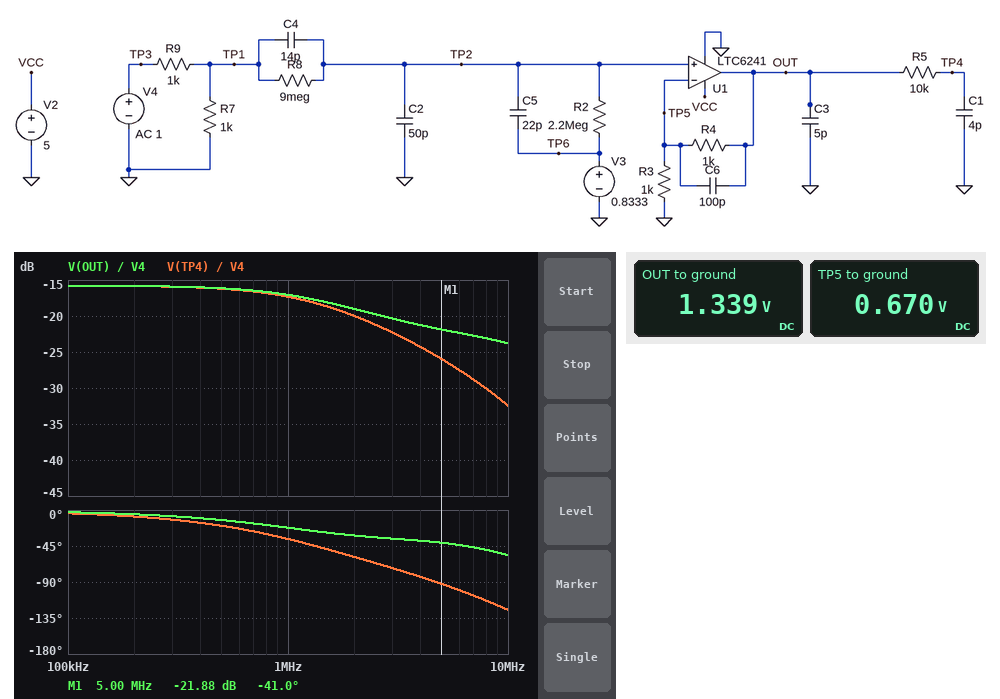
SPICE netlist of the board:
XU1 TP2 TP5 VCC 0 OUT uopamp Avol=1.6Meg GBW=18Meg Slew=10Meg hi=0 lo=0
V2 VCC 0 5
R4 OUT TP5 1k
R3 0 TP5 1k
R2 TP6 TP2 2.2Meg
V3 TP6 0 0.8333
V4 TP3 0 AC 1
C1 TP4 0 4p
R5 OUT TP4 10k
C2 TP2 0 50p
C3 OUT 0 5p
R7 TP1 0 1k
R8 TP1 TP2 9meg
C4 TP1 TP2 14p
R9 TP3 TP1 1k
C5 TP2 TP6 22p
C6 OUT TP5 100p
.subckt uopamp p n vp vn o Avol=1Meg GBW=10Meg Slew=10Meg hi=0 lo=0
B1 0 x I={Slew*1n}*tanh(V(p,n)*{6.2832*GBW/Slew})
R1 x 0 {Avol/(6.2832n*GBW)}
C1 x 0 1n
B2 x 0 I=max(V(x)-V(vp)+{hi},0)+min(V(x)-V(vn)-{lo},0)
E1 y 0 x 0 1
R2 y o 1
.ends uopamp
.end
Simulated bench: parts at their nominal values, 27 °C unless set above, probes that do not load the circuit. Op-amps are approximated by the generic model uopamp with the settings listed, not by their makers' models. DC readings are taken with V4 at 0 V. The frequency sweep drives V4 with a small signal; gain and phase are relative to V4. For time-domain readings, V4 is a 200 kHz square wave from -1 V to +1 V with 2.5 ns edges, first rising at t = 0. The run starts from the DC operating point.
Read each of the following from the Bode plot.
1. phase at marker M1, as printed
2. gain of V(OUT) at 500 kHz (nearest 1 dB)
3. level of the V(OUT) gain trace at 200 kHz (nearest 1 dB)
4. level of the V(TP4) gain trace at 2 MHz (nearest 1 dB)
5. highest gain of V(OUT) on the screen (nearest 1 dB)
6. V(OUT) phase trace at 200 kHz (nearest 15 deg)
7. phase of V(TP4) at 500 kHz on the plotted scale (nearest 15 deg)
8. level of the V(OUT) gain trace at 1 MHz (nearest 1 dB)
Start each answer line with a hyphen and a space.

- -41.0 deg
- -16 dB
- -16 dB
- -20 dB
- -16 dB
- 0 deg
- -15 deg
- -17 dB
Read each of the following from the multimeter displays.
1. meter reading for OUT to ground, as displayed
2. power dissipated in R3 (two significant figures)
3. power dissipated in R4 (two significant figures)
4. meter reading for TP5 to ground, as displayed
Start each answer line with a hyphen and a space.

- 1.339 V
- 450 µW
- 450 µW
- 0.670 V
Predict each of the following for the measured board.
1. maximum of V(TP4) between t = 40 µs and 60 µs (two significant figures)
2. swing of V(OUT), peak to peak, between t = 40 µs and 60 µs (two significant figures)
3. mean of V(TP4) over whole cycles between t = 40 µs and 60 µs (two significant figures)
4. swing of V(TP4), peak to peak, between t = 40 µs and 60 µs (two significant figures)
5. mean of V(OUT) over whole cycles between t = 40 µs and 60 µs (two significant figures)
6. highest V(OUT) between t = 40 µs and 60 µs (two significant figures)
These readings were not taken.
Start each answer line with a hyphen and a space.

- 1.5 V
- 330 mV
- 1.3 V
- 330 mV
- 1.3 V
- 1.5 V
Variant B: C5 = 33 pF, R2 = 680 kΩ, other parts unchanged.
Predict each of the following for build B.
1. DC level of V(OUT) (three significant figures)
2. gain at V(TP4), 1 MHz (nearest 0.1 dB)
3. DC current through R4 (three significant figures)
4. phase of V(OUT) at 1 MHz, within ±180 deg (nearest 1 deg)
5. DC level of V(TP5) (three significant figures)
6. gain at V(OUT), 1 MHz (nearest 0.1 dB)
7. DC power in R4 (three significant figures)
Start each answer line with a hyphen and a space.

- 1.55 V
- -18.4 dB
- 775 µA
- -22 deg
- 775 mV
- -18.1 dB
- 600 µW
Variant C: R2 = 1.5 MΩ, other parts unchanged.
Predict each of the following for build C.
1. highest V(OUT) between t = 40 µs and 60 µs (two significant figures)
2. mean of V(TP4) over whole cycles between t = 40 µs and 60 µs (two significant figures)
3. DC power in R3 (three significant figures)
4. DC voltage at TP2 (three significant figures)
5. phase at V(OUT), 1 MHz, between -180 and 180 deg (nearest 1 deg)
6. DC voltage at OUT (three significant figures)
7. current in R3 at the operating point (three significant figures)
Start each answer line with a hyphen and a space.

- 1.6 V
- 1.4 V
- 510 µW
- 714 mV
- -22 deg
- 1.43 V
- 714 µA
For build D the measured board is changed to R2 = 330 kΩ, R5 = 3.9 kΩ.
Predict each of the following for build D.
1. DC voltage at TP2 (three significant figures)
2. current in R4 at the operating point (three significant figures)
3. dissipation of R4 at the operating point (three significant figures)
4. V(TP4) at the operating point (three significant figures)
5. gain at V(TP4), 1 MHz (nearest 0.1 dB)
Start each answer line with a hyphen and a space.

- 804 mV
- 804 µA
- 646 µW
- 1.61 V
- -17.1 dB
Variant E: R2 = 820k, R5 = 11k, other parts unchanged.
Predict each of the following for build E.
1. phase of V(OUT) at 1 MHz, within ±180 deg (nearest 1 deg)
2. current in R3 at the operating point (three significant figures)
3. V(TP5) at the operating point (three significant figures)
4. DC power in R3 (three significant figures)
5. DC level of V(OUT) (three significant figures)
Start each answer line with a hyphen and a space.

- -22 deg
- 764 µA
- 764 mV
- 583 µW
- 1.53 V
